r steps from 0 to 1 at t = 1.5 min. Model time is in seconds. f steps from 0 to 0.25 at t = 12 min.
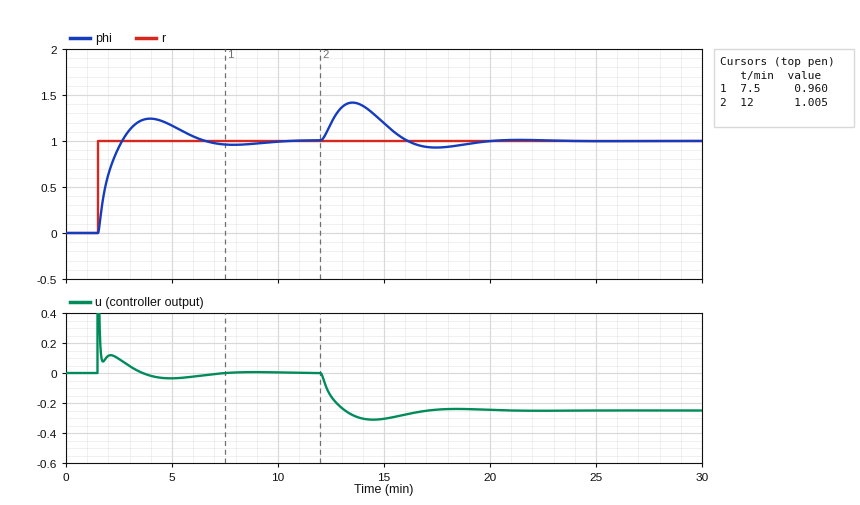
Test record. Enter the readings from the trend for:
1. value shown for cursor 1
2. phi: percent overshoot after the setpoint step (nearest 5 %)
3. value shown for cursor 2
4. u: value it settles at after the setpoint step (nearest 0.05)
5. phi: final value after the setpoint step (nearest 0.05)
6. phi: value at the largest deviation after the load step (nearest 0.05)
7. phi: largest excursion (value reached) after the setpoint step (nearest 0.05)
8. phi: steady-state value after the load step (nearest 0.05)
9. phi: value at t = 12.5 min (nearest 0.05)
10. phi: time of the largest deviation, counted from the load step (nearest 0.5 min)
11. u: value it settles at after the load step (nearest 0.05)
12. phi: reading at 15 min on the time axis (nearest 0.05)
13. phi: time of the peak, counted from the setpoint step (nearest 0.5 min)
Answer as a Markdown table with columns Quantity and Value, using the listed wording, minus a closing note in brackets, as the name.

| Quantity | Value |
|---|---|
| value shown for cursor 1 | 0.960 |
| phi: percent overshoot after the setpoint step | 25 % |
| value shown for cursor 2 | 1.005 |
| u: value it settles at after the setpoint step | 0.00 |
| phi: final value after the setpoint step | 1.00 |
| phi: value at the largest deviation after the load step | 1.40 |
| phi: largest excursion (value reached) after the setpoint step | 1.25 |
| phi: steady-state value after the load step | 1.00 |
| phi: value at t = 12.5 min | 1.20 |
| phi: time of the largest deviation, counted from the load step | 1.5 min |
| u: value it settles at after the load step | -0.25 |
| phi: reading at 15 min on the time axis | 1.20 |
| phi: time of the peak, counted from the setpoint step | 2.5 min |
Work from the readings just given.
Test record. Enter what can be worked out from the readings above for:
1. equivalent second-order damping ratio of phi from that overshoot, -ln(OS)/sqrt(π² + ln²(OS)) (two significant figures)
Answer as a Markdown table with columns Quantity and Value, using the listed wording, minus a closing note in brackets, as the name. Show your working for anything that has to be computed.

| Quantity | Value |
|---|---|
| equivalent second-order damping ratio of phi from that overshoot, -ln(OS)/sqrt(π² + ln²(OS)) | ln(0.25) = -1.386; 1.386 / sqrt(9.870 + 1.922) = 0.40 |
